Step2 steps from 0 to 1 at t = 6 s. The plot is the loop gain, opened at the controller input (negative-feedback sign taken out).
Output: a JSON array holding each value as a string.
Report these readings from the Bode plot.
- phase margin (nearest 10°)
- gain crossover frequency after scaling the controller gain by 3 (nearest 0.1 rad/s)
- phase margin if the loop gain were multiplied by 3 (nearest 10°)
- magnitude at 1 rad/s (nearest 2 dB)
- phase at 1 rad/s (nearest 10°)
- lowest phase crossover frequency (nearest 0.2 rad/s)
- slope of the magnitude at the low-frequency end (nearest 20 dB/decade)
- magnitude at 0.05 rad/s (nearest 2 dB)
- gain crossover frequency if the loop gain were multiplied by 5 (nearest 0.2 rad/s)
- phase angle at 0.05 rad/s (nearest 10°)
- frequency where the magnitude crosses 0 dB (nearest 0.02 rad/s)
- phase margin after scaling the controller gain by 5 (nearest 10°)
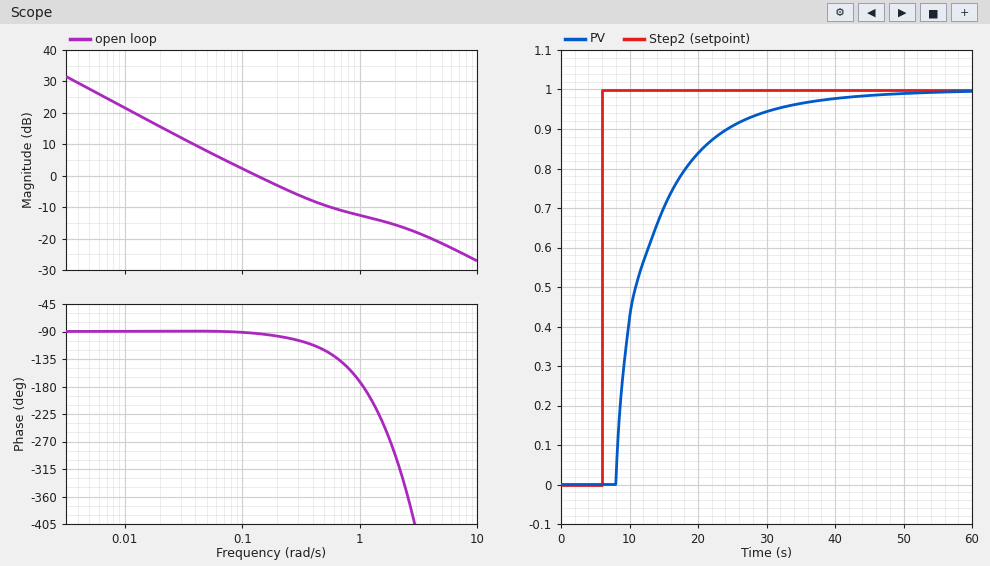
["90°", "0.5 rad/s", "60°", "-12 dB", "-170°", "1.0 rad/s", "-20 dB/decade", "8 dB", "1.4 rad/s", "-90°", "0.14 rad/s", "-40°"]
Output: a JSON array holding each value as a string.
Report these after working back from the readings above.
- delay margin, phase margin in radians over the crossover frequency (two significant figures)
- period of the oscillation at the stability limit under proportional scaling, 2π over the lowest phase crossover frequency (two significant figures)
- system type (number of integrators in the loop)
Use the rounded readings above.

["11 s", "6.3 s", "1"]
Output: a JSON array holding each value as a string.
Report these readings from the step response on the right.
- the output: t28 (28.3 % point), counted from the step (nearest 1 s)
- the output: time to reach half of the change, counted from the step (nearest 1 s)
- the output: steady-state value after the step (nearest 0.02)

["3 s", "5 s", "1.00"]
